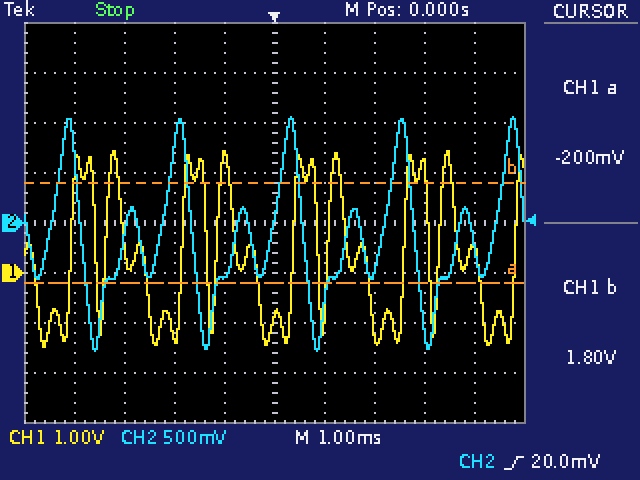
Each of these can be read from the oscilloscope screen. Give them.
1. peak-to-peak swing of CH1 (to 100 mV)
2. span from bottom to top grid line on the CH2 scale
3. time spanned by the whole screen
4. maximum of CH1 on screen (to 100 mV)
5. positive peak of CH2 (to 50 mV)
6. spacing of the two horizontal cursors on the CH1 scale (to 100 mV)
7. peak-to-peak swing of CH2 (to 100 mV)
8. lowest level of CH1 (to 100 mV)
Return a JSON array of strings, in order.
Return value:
["3.9 V", "4 V", "10 ms", "2.4 V", "1.05 V", "2.0 V", "2.30 V", "-1.5 V"]
